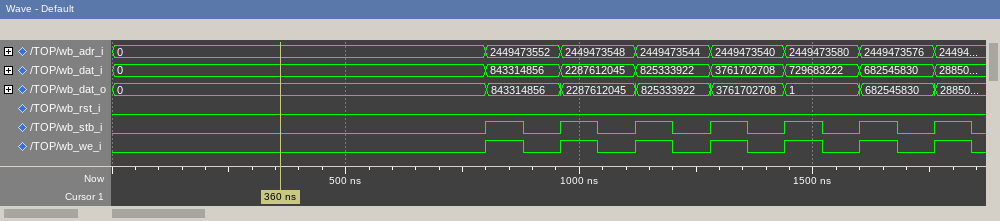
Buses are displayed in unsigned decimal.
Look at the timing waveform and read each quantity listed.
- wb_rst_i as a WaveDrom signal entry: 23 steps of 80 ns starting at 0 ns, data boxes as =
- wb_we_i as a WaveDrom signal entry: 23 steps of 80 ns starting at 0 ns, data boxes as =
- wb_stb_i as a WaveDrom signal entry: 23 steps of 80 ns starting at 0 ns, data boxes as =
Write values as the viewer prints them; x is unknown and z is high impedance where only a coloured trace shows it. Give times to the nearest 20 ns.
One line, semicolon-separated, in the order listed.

{name: 'wb_rst_i', wave: '0......................'}; {name: 'wb_we_i', wave: '0.........1010101010101'}; {name: 'wb_stb_i', wave: '0.........1010101010101'}
